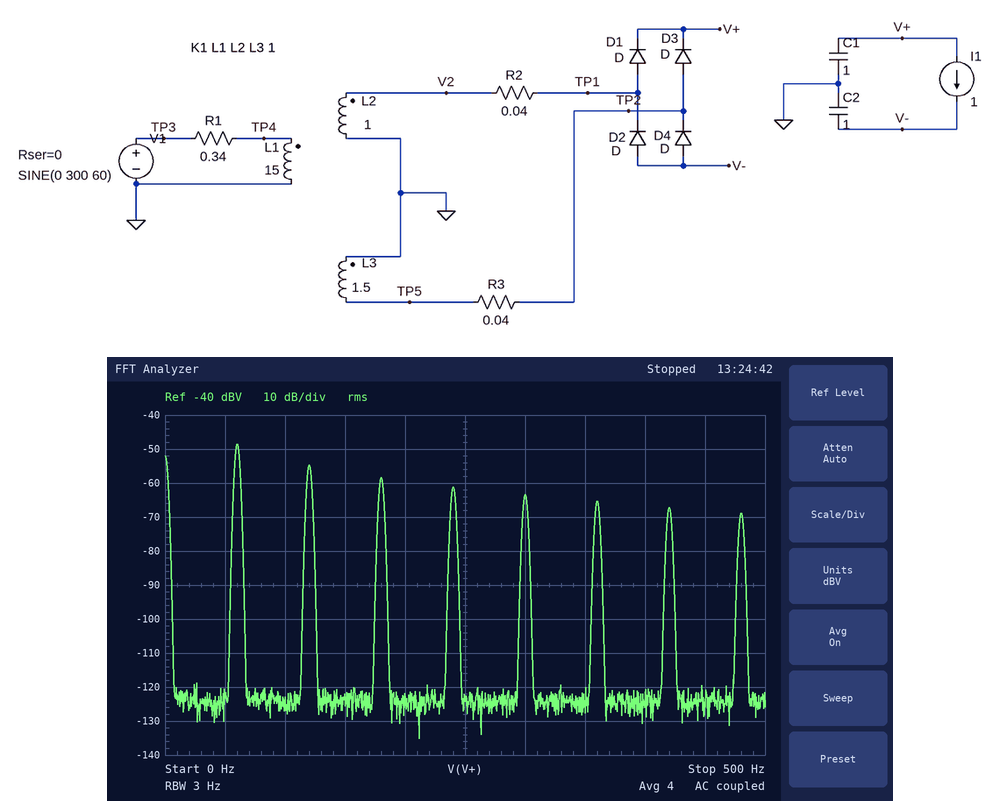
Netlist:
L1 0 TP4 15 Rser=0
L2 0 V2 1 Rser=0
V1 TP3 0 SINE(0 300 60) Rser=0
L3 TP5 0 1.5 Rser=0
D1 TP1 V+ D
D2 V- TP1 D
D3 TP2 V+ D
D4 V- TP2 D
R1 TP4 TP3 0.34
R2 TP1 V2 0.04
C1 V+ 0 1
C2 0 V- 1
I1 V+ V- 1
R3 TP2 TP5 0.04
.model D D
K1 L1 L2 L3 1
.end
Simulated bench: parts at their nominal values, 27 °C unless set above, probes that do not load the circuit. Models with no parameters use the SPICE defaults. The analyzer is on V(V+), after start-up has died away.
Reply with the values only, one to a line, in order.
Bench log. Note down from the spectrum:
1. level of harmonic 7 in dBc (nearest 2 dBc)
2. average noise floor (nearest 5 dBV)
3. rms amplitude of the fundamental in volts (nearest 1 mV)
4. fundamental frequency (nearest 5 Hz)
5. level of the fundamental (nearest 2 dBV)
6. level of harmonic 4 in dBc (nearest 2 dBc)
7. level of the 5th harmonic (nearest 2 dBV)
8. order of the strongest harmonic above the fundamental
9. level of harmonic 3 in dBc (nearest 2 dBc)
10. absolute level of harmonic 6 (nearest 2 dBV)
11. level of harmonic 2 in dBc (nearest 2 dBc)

-18 dBc
-125 dBV
4 mV
60 Hz
-48 dBV
-12 dBc
-64 dBV
2
-10 dBc
-66 dBV
-6 dBc
